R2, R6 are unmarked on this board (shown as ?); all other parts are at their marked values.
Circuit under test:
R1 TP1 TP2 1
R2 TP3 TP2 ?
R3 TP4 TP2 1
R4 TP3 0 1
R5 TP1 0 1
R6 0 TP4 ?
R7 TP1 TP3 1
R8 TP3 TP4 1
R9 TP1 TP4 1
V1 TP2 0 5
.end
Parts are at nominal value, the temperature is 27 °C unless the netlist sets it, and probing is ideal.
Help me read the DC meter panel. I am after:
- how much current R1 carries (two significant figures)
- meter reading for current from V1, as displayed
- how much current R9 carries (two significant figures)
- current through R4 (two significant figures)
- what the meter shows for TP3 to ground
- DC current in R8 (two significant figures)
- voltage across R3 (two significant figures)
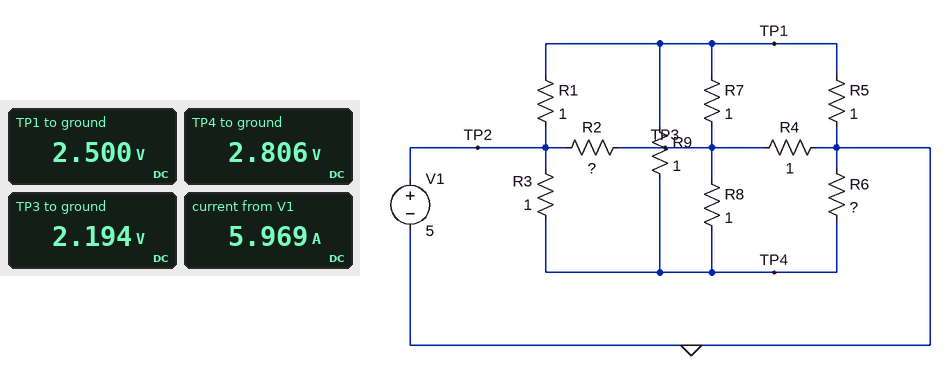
2.5 A
5.969 A
310 mA
2.2 A
2.194 V
610 mA
2.2 V
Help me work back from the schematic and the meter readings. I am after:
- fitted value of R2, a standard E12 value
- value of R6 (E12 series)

2.2 Ω
2.2 Ω
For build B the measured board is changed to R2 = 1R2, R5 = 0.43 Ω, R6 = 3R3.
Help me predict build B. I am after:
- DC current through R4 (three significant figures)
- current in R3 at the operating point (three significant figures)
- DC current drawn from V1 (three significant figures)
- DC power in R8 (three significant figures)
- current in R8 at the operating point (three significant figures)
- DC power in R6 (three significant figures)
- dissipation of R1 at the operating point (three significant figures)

2.31 A
2.21 A
7.56 A
229 mW
478 mA
2.35 W
9.64 W
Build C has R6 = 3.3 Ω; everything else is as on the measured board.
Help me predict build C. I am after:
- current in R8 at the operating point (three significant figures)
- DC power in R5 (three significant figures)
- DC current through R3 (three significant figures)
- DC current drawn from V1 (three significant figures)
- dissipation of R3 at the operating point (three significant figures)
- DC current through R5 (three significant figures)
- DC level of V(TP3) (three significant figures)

713 mA
6.54 W
2.03 A
5.72 A
4.11 W
2.56 A
2.26 V
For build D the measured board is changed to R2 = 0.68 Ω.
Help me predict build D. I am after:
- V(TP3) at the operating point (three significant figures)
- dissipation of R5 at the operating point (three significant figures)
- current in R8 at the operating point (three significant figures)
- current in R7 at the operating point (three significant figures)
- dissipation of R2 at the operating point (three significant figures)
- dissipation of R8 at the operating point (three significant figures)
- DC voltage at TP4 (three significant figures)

2.96 V
7.65 W
146 mA
192 mA
6.13 W
21.4 mW
3.10 V
